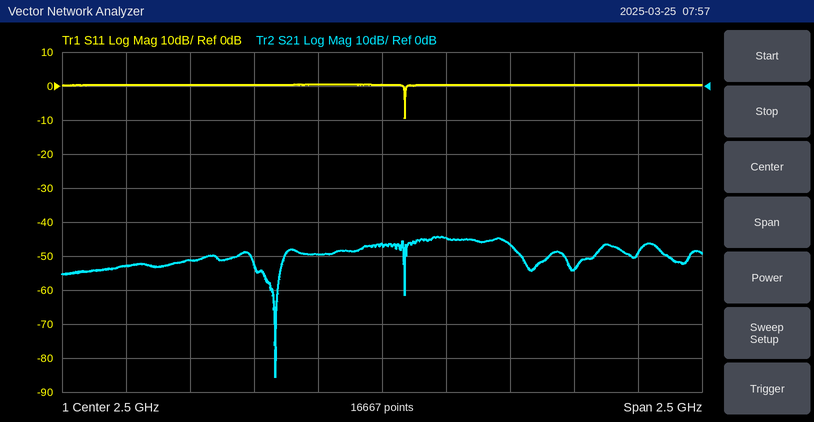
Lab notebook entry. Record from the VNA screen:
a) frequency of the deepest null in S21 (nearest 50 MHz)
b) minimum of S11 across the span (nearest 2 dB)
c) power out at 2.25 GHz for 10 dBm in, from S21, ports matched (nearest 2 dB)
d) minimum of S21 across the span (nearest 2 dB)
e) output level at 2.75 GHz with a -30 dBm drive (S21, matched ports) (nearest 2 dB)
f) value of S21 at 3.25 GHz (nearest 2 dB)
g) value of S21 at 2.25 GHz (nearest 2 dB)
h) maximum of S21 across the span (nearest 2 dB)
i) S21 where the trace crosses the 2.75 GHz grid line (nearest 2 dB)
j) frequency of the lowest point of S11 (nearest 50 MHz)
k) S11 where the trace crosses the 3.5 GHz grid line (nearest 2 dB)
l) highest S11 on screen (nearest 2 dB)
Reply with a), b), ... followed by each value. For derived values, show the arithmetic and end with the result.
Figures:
a) 2.10 GHz
b) -10 dB
c) 10 dBm + (-50 dB) = -40 dBm
d) -86 dB
e) -30 dBm + (-44 dB) = -74 dBm
f) -54 dB
g) -50 dB
h) -44 dB
i) -44 dB
j) 2.60 GHz
k) 0 dB
l) 0 dB
